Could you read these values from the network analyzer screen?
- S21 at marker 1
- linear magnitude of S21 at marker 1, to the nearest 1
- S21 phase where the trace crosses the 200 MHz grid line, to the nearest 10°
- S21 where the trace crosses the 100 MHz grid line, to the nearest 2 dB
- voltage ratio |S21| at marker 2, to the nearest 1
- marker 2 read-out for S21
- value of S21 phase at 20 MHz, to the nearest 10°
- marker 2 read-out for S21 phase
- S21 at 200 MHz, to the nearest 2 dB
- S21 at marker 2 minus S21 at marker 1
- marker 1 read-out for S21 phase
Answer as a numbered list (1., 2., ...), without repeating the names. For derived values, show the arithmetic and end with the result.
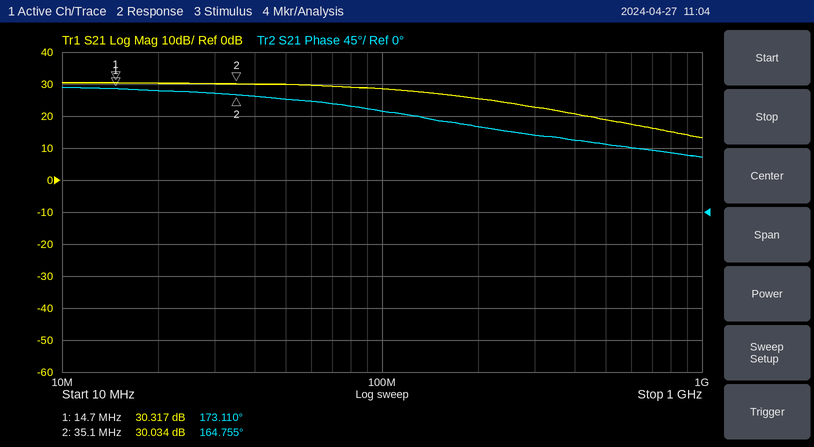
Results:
1. 30.317 dB
2. 10^(30.317/20) ≈ 33
3. 120°
4. 28 dB
5. 10^(30.034/20) ≈ 32
6. 30.034 dB
7. 170°
8. 164.755°
9. 26 dB
10. 30.034 − (30.317) = -0.283 dB
11. 173.110°
